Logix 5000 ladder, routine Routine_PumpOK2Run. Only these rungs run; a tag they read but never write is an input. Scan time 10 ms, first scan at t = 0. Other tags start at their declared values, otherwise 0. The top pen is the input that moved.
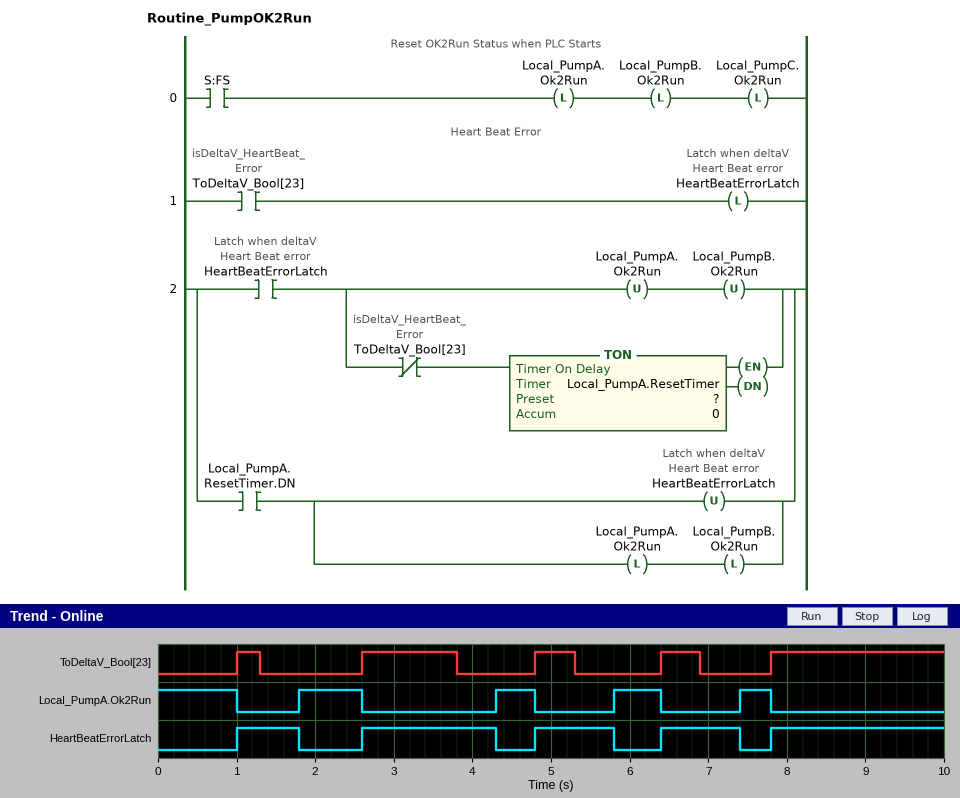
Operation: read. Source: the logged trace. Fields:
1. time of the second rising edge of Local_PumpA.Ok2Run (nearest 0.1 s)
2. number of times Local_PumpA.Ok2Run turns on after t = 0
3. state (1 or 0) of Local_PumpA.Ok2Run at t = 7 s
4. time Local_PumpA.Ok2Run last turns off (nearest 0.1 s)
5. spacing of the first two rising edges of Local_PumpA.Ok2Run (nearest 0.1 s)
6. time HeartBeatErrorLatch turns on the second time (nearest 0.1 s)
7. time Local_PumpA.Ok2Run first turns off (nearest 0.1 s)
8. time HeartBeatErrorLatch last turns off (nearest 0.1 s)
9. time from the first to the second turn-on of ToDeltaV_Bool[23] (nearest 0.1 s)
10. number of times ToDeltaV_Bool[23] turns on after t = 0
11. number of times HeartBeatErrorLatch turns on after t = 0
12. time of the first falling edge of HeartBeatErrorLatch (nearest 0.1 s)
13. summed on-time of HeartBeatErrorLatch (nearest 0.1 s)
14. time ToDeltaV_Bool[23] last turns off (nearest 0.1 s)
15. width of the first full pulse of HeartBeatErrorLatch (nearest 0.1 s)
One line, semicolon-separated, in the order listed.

4.3 s; 4; 0; 7.8 s; 2.5 s; 2.6 s; 1.0 s; 7.4 s; 1.6 s; 5; 5; 1.8 s; 6.7 s; 6.9 s; 0.8 s
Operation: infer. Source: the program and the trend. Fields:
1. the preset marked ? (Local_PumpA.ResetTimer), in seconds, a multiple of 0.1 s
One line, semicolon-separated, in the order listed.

0.5 s
